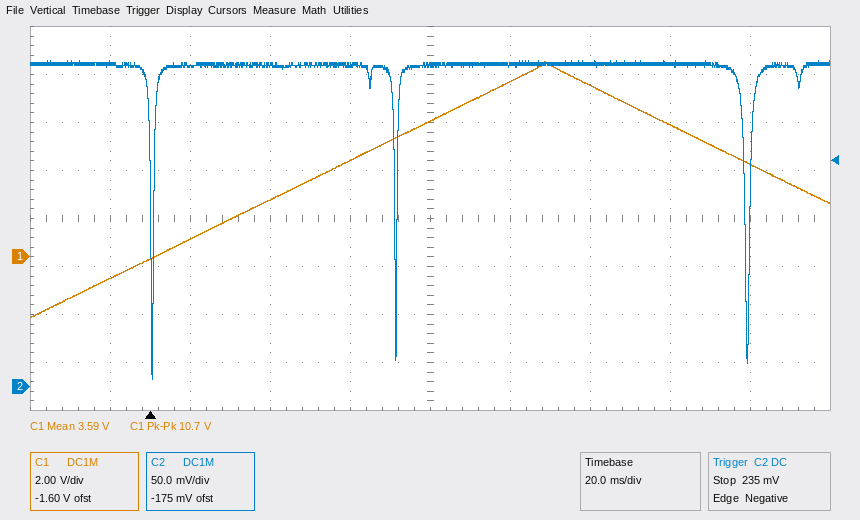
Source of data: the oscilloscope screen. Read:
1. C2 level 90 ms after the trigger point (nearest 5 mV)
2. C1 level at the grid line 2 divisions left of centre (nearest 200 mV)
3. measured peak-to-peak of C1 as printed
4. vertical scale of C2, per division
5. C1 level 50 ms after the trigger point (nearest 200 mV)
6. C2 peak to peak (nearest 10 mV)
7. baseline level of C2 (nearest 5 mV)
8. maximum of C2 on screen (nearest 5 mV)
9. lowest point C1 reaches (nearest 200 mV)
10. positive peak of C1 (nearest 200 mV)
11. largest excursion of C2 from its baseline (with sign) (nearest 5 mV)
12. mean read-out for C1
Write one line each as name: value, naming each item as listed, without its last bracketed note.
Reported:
C2 level 90 ms after the trigger point: 335 mV
C1 level at the grid line 2 divisions left of centre: 2.4 V
measured peak-to-peak of C1 as printed: 10.7 V
vertical scale of C2, per division: 50 mV
C1 level 50 ms after the trigger point: 4.0 V
C2 peak to peak: 330 mV
baseline level of C2: 335 mV
maximum of C2 on screen: 340 mV
lowest point C1 reaches: -2.6 V
positive peak of C1: 8.2 V
largest excursion of C2 from its baseline (with sign): -330 mV
mean read-out for C1: 3.59 V
